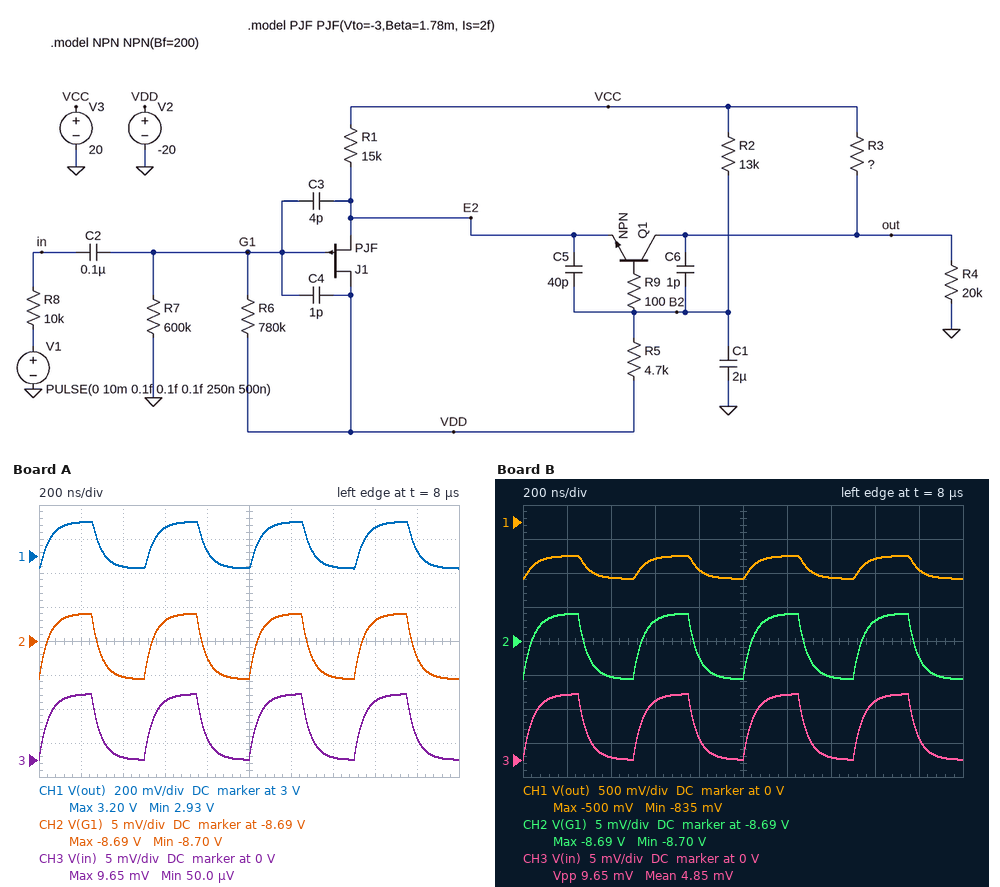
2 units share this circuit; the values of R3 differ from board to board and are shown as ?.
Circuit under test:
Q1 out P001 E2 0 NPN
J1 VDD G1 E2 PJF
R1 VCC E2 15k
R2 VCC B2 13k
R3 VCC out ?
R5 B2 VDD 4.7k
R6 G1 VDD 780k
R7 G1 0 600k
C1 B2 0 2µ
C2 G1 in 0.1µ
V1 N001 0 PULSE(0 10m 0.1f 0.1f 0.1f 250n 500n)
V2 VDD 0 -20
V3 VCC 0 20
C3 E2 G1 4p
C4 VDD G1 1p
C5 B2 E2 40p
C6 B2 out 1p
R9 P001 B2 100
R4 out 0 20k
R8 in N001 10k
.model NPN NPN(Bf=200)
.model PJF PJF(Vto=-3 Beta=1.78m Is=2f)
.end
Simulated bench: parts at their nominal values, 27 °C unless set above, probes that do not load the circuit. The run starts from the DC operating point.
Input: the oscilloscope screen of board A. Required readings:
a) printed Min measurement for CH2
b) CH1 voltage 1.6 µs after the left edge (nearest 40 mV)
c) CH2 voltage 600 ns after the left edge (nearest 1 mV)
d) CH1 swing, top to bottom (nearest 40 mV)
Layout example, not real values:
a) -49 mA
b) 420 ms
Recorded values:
a) -8.70 V
b) 3.16 V
c) -8.687 V
d) 280 mV
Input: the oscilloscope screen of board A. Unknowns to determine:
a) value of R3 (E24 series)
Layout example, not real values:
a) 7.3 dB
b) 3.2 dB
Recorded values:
a) 8.2 kΩ
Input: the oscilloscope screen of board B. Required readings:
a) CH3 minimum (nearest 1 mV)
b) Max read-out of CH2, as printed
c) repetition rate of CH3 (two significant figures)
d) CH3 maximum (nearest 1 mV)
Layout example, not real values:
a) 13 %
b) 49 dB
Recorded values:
a) 0 V
b) -8.69 V
c) 2.0 MHz
d) 10 mV
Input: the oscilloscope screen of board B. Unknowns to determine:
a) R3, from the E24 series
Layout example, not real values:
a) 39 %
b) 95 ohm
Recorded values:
a) 11 kΩ
